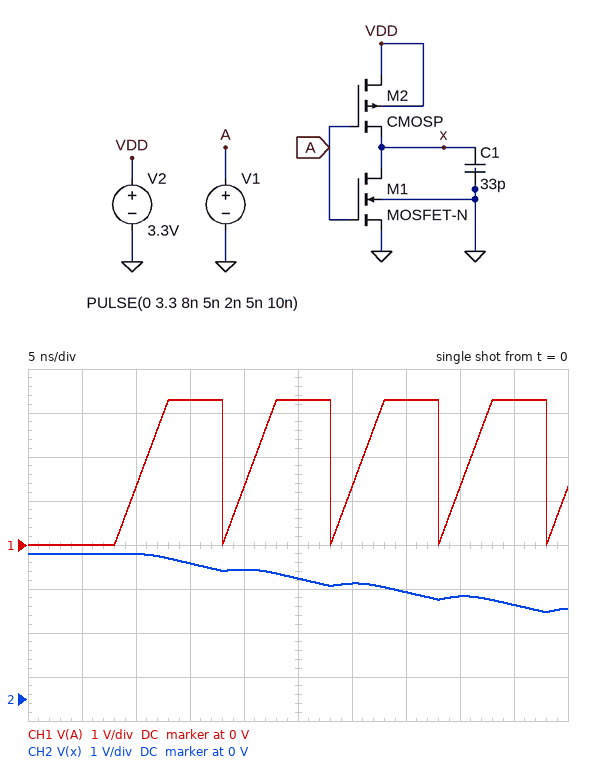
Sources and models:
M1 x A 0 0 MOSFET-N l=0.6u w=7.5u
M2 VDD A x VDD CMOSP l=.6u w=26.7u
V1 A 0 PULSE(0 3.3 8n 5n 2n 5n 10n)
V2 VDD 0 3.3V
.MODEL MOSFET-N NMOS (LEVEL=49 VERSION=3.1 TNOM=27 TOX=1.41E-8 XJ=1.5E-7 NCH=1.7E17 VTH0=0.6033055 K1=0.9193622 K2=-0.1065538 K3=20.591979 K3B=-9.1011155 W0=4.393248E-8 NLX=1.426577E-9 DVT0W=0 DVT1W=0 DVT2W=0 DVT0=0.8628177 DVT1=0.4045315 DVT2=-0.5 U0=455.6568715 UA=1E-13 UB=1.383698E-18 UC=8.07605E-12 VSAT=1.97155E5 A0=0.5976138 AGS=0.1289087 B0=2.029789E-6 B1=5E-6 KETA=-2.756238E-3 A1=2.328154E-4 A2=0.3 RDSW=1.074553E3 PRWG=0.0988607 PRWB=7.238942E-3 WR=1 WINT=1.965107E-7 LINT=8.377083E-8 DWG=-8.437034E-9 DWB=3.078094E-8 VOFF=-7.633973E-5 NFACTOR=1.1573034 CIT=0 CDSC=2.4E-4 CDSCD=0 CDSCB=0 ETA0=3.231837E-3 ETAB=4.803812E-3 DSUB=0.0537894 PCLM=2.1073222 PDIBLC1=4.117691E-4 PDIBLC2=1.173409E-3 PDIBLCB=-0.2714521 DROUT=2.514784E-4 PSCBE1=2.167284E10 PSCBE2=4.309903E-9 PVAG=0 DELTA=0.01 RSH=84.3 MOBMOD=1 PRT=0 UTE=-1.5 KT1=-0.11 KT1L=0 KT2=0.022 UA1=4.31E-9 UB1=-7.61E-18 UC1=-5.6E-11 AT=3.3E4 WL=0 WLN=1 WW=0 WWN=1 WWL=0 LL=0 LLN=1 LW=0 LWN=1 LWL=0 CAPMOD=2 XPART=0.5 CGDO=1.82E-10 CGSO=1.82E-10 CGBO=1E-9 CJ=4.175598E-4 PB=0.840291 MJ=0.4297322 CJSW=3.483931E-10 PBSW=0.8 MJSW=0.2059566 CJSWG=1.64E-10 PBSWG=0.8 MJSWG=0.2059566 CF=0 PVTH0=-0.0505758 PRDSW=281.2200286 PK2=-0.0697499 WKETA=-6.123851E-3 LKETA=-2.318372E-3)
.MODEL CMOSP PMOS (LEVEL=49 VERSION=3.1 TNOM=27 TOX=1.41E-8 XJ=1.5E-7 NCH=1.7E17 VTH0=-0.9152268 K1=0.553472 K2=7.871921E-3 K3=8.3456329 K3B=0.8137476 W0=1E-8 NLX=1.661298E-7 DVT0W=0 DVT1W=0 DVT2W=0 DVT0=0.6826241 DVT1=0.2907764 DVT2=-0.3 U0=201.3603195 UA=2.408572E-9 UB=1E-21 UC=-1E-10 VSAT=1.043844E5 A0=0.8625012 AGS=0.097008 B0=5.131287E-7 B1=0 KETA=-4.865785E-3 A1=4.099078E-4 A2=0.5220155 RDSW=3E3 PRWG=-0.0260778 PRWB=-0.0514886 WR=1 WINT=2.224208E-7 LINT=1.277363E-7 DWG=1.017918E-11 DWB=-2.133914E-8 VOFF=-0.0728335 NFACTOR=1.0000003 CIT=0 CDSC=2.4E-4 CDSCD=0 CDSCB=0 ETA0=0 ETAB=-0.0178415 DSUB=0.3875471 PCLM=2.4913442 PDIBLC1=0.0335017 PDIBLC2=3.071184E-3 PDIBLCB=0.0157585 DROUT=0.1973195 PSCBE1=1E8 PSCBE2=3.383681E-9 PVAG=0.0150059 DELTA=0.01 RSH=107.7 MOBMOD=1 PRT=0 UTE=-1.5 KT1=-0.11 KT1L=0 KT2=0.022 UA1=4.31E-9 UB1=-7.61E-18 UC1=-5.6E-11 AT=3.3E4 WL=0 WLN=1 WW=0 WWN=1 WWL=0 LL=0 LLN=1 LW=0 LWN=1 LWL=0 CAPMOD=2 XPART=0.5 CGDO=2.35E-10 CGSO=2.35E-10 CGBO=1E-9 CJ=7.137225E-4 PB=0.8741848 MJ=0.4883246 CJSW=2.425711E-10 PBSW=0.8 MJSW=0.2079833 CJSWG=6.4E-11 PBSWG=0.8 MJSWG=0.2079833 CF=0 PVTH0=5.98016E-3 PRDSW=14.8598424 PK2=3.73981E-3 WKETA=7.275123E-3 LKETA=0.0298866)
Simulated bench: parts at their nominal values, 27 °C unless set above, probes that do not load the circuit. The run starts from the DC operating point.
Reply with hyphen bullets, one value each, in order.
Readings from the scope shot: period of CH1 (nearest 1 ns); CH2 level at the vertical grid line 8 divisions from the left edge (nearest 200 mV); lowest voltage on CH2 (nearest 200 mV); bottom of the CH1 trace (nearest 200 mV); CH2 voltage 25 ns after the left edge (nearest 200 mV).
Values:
- 10 ns
- 2.4 V
- 2.0 V
- 0 V
- 2.8 V
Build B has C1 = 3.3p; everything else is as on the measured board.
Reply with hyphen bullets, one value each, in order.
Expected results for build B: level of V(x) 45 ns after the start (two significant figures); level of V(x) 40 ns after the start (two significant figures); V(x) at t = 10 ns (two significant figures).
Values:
- 220 mV
- 1.1 V
- 3.3 V
